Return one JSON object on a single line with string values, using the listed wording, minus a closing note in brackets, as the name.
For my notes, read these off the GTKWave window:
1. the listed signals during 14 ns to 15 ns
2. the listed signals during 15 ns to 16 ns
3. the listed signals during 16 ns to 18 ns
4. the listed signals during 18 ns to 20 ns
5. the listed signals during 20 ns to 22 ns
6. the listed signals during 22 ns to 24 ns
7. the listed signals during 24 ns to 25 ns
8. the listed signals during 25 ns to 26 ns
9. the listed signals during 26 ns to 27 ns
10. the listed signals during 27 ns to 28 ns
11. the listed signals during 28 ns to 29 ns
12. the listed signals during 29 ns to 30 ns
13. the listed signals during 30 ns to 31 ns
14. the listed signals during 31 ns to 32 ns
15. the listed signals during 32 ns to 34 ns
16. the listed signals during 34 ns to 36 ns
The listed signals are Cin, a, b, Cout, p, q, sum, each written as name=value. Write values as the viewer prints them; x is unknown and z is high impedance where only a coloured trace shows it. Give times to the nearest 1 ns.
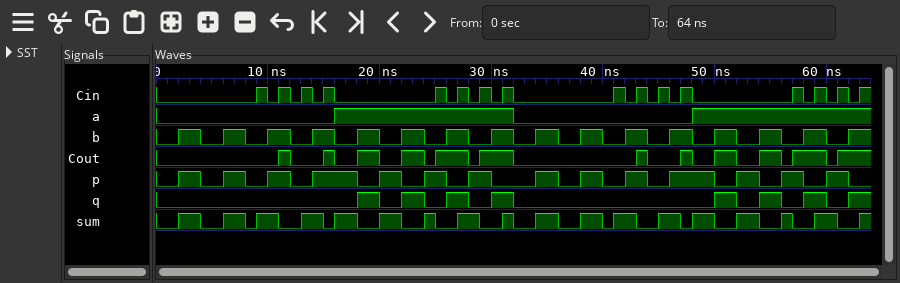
{"the listed signals during 14 ns to 15 ns": "Cin=0, a=0, b=1, Cout=0, p=1, q=0, sum=1", "the listed signals during 15 ns to 16 ns": "Cin=1, a=0, b=1, Cout=1, p=1, q=0, sum=0", "the listed signals during 16 ns to 18 ns": "Cin=0, a=1, b=0, Cout=0, p=1, q=0, sum=1", "the listed signals during 18 ns to 20 ns": "Cin=0, a=1, b=1, Cout=1, p=0, q=1, sum=0", "the listed signals during 20 ns to 22 ns": "Cin=0, a=1, b=0, Cout=0, p=1, q=0, sum=1", "the listed signals during 22 ns to 24 ns": "Cin=0, a=1, b=1, Cout=1, p=0, q=1, sum=0", "the listed signals during 24 ns to 25 ns": "Cin=0, a=1, b=0, Cout=0, p=1, q=0, sum=1", "the listed signals during 25 ns to 26 ns": "Cin=1, a=1, b=0, Cout=1, p=1, q=0, sum=0", "the listed signals during 26 ns to 27 ns": "Cin=0, a=1, b=1, Cout=1, p=0, q=1, sum=0", "the listed signals during 27 ns to 28 ns": "Cin=1, a=1, b=1, Cout=1, p=0, q=1, sum=1", "the listed signals during 28 ns to 29 ns": "Cin=0, a=1, b=0, Cout=0, p=1, q=0, sum=1", "the listed signals during 29 ns to 30 ns": "Cin=1, a=1, b=0, Cout=1, p=1, q=0, sum=0", "the listed signals during 30 ns to 31 ns": "Cin=0, a=1, b=1, Cout=1, p=0, q=1, sum=0", "the listed signals during 31 ns to 32 ns": "Cin=1, a=1, b=1, Cout=1, p=0, q=1, sum=1", "the listed signals during 32 ns to 34 ns": "Cin=0, a=0, b=0, Cout=0, p=0, q=0, sum=0", "the listed signals during 34 ns to 36 ns": "Cin=0, a=0, b=1, Cout=0, p=1, q=0, sum=1"}
